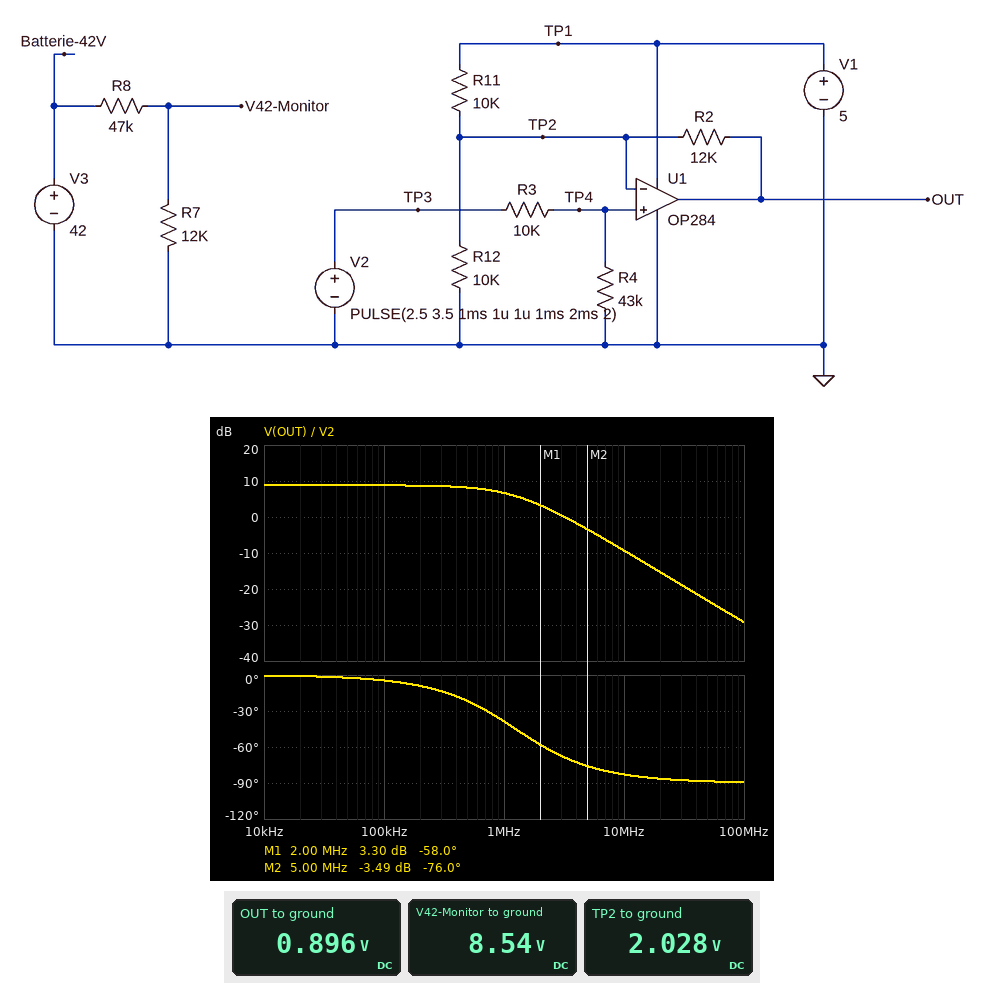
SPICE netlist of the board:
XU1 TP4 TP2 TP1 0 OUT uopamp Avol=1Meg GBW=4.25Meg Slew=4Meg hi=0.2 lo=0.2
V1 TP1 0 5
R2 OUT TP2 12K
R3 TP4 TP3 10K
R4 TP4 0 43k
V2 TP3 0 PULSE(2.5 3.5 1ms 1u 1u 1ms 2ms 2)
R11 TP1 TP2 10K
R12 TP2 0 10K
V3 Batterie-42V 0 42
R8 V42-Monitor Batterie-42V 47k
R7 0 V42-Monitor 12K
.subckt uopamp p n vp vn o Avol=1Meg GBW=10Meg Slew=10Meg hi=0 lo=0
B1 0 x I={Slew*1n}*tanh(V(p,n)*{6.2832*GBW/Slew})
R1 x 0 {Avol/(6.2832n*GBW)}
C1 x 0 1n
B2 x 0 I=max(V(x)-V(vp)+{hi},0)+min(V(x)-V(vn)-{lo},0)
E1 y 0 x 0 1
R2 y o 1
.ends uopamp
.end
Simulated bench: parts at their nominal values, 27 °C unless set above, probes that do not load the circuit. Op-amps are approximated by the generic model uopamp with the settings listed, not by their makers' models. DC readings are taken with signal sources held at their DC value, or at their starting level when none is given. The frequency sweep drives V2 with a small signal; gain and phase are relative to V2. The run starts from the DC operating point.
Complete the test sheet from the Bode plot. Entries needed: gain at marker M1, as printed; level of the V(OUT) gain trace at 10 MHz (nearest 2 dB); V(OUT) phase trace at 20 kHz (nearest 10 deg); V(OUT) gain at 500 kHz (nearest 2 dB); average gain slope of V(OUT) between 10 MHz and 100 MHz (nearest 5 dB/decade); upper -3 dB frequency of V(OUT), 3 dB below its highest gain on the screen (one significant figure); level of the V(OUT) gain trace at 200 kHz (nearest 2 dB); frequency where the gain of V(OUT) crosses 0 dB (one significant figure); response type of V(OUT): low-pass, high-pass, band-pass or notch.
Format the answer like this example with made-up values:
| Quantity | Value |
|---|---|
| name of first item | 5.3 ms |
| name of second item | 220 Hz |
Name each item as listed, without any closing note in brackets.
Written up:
| Quantity | Value |
|---|---|
| gain at marker M1, as printed | 3.30 dB |
| level of the V(OUT) gain trace at 10 MHz | -10 dB |
| V(OUT) phase trace at 20 kHz | 0 deg |
| V(OUT) gain at 500 kHz | 8 dB |
| average gain slope of V(OUT) between 10 MHz and 100 MHz | -20 dB/decade |
| upper -3 dB frequency of V(OUT), 3 dB below its highest gain on the screen | 1 MHz |
| level of the V(OUT) gain trace at 200 kHz | 8 dB |
| frequency where the gain of V(OUT) crosses 0 dB | 3 MHz |
| response type of V(OUT): low-pass, high-pass, band-pass or notch | low-pass |
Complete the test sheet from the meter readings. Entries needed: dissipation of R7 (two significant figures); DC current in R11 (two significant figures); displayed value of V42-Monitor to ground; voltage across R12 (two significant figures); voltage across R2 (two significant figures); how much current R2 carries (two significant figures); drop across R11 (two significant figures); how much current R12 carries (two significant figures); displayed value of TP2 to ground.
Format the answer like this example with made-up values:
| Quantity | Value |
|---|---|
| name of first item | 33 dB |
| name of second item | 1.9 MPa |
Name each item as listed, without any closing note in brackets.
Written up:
| Quantity | Value |
|---|---|
| dissipation of R7 | 6.1 mW |
| DC current in R11 | 300 µA |
| displayed value of V42-Monitor to ground | 8.54 V |
| voltage across R12 | 2.0 V |
| voltage across R2 | 1.1 V |
| how much current R2 carries | 94 µA |
| drop across R11 | 3.0 V |
| how much current R12 carries | 200 µA |
| displayed value of TP2 to ground | 2.028 V |
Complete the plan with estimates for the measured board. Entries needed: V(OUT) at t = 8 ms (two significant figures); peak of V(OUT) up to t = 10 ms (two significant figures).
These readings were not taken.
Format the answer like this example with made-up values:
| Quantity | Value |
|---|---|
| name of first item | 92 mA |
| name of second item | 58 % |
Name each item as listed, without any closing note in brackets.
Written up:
| Quantity | Value |
|---|---|
| V(OUT) at t = 8 ms | 900 mV |
| peak of V(OUT) up to t = 10 ms | 3.7 V |
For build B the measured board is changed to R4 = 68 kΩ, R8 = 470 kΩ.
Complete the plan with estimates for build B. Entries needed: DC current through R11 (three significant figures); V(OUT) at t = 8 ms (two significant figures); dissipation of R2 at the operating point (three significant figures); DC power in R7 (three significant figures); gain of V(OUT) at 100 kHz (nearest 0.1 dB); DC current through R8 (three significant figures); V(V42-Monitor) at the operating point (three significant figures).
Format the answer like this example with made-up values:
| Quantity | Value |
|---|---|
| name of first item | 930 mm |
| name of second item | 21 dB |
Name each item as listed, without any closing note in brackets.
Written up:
| Quantity | Value |
|---|---|
| DC current through R11 | 282 µA |
| V(OUT) at t = 8 ms | 1.4 V |
| dissipation of R2 at the operating point | 49.3 µW |
| DC power in R7 | 91.1 µW |
| gain of V(OUT) at 100 kHz | 9.4 dB |
| DC current through R8 | 87.1 µA |
| V(V42-Monitor) at the operating point | 1.05 V |
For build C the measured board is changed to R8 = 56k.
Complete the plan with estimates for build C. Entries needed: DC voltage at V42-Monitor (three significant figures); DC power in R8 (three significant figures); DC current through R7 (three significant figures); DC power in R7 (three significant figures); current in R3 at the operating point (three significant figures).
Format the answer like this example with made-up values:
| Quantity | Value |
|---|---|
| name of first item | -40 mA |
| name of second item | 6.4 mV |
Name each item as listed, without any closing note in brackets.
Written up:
| Quantity | Value |
|---|---|
| DC voltage at V42-Monitor | 7.41 V |
| DC power in R8 | 21.4 mW |
| DC current through R7 | 618 µA |
| DC power in R7 | 4.58 mW |
| current in R3 at the operating point | 47.2 µA |
